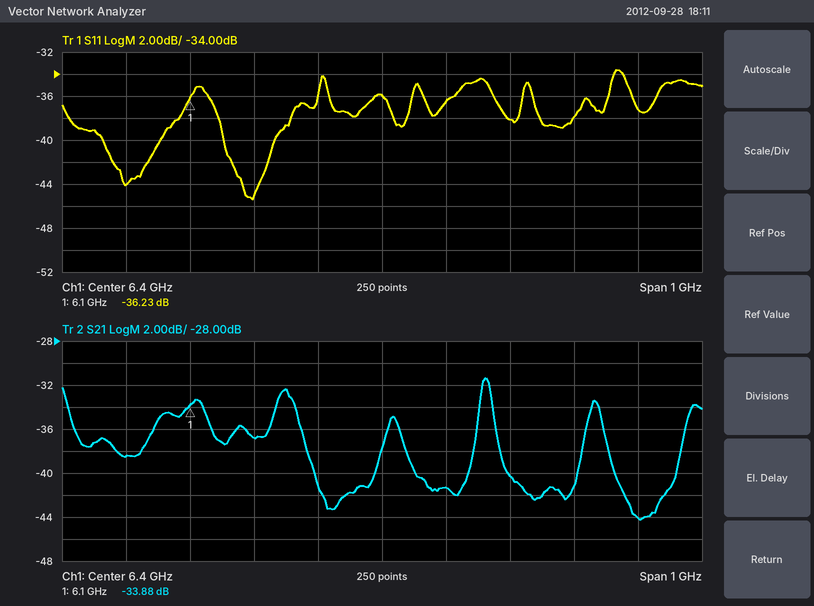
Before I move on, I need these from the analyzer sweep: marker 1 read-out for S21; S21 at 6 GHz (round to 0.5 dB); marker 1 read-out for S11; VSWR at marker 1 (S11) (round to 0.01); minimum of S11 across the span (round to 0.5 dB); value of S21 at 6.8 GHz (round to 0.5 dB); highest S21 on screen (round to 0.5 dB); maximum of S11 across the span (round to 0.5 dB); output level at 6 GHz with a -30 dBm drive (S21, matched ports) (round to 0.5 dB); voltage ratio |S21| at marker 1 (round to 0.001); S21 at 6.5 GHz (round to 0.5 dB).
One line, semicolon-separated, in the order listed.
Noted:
-33.88 dB; -38.5 dB; -36.23 dB; 1.03; -45.5 dB; -44.0 dB; -31.5 dB; -33.5 dB; -68.5 dBm; 0.020; -41.5 dB
